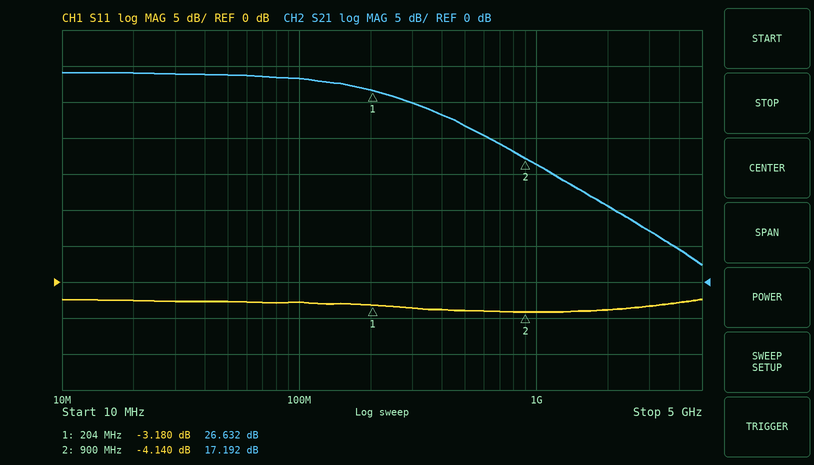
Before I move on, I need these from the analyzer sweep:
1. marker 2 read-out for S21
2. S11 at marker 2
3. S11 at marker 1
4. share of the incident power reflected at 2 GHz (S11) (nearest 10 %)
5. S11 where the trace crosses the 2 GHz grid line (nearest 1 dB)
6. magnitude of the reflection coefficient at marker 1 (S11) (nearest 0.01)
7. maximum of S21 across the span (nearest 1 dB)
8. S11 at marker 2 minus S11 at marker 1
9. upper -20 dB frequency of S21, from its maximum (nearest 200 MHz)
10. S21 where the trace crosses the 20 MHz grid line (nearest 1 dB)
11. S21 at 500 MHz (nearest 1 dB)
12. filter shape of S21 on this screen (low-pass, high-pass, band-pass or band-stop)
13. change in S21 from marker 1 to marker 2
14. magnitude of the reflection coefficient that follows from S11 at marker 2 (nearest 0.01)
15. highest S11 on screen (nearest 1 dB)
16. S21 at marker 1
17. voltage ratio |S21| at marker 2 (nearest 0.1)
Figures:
17.192 dB
-4.140 dB
-3.180 dB
40 %
-4 dB
0.69
29 dB
-0.960 dB
2.4 GHz
29 dB
22 dB
low-pass
-9.440 dB
0.62
-2 dB
26.632 dB
7.2
